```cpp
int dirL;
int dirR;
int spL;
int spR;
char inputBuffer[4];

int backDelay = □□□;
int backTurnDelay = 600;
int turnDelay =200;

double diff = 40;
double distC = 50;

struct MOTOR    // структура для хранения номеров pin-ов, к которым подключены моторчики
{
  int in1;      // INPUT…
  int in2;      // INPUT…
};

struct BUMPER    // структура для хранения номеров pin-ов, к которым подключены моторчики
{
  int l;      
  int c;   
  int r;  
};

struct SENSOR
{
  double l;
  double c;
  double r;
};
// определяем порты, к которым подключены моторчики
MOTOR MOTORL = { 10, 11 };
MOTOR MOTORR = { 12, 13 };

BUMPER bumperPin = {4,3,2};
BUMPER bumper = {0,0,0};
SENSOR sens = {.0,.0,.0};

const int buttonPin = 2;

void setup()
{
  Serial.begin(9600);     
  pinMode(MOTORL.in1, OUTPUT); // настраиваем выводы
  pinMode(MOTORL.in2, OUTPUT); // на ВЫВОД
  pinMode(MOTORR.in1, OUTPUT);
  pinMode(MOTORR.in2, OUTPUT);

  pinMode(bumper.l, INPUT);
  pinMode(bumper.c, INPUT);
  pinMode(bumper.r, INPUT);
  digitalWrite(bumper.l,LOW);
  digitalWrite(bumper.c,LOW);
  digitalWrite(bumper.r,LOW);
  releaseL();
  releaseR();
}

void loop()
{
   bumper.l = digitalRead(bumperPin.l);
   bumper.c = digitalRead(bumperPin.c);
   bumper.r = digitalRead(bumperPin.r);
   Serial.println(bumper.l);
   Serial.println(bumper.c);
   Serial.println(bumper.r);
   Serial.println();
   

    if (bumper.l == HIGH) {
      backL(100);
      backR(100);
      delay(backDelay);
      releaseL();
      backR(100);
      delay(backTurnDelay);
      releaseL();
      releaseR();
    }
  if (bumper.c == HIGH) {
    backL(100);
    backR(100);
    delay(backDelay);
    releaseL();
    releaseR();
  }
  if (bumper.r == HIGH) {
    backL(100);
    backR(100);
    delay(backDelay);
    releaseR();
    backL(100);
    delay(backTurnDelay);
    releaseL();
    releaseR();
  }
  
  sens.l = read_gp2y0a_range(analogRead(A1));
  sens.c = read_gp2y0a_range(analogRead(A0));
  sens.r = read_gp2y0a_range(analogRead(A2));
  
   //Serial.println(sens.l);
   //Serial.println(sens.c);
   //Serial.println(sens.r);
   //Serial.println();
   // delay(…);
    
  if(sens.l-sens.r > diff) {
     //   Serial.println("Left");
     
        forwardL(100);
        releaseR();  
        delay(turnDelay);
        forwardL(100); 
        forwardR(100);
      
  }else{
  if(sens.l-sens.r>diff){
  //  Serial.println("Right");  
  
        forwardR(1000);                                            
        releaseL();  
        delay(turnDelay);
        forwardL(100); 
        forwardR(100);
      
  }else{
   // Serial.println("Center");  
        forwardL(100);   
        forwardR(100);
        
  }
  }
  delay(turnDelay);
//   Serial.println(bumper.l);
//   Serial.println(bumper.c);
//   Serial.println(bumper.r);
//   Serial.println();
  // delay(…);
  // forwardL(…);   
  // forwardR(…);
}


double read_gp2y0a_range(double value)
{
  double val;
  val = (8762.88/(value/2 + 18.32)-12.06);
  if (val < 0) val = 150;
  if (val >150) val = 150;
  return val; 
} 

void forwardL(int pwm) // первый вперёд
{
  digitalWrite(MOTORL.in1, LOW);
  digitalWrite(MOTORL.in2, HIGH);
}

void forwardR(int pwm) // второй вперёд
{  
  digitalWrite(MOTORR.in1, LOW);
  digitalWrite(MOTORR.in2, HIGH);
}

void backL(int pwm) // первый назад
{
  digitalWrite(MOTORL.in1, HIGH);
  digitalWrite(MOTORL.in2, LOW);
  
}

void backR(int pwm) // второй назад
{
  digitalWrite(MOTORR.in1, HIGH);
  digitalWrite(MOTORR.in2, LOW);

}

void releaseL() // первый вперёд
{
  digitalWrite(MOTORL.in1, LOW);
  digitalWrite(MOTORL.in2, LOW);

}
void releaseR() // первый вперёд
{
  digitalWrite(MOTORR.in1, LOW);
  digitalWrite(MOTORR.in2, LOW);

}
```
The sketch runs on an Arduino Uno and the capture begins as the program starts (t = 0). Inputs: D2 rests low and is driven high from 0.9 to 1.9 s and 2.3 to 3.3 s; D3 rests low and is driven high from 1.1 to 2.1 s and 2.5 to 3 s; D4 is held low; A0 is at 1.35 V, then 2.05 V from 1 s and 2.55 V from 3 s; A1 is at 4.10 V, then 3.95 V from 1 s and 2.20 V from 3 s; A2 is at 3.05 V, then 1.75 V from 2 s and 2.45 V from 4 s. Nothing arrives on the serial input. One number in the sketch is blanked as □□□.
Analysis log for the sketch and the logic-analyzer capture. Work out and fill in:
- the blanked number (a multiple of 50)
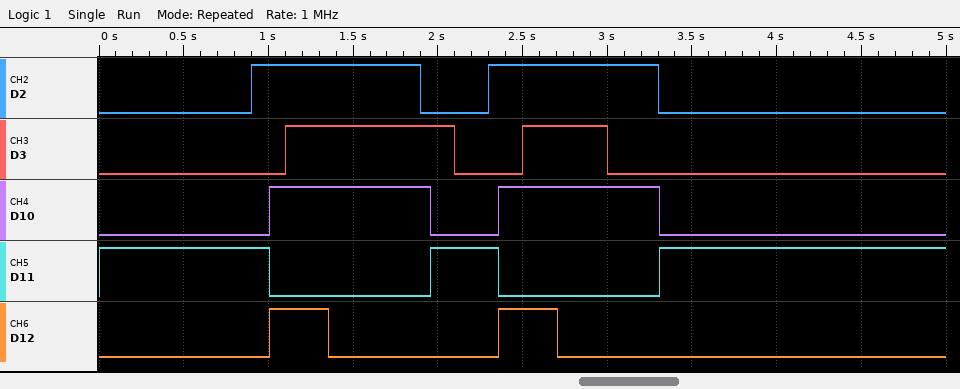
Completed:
350
